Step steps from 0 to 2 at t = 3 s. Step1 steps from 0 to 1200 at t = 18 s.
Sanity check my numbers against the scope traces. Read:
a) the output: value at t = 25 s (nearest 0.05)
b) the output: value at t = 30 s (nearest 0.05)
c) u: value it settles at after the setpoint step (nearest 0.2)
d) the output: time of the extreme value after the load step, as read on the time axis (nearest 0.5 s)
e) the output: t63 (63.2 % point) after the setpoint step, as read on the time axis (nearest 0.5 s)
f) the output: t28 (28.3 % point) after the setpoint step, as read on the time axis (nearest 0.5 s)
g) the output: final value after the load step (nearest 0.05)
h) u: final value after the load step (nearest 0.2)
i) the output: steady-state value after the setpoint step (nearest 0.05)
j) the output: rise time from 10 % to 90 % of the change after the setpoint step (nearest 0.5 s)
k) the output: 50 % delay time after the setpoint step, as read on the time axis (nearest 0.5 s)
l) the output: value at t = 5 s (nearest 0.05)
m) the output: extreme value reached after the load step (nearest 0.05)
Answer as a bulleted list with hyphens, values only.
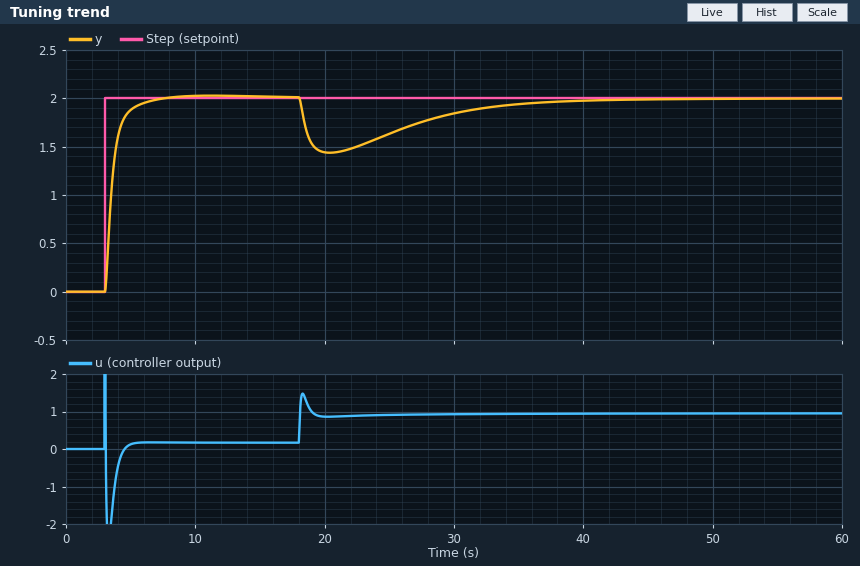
- 1.65
- 1.85
- 0.2
- 20.5 s
- 3.5 s
- 3.5 s
- 2.00
- 1.0
- 2.00
- 1.5 s
- 3.5 s
- 1.90
- 1.45
